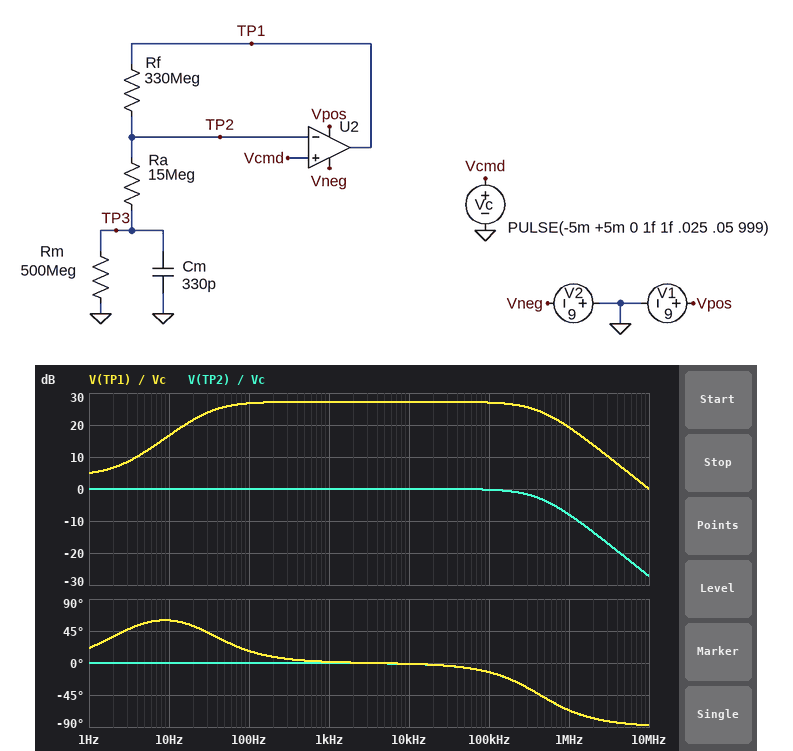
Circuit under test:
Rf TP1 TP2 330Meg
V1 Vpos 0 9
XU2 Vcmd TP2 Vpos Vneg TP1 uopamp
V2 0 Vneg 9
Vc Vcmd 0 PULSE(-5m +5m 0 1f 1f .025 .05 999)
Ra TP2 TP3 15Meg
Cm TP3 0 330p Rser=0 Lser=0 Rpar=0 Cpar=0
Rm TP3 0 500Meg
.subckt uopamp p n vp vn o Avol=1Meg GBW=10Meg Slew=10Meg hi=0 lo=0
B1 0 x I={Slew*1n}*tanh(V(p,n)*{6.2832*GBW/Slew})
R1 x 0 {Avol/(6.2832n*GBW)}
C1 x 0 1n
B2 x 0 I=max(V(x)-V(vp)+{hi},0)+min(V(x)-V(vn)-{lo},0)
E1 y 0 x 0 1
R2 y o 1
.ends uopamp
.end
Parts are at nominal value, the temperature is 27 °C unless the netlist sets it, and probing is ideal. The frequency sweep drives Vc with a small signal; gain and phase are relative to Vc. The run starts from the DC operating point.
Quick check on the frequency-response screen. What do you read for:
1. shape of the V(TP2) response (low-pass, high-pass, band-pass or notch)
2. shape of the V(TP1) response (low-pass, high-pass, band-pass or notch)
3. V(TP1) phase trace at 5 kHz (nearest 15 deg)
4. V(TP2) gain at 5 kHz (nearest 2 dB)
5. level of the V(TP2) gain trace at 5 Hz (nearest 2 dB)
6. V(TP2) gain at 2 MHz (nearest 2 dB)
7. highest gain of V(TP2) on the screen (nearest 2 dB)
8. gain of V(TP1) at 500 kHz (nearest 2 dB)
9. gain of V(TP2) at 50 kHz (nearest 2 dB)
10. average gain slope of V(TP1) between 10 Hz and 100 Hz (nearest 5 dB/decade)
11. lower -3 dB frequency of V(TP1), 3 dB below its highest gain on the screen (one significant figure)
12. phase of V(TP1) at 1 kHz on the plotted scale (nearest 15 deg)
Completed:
low-pass
band-pass
0 deg
0 dB
0 dB
-14 dB
0 dB
24 dB
0 dB
10 dB/decade
30 Hz
0 deg
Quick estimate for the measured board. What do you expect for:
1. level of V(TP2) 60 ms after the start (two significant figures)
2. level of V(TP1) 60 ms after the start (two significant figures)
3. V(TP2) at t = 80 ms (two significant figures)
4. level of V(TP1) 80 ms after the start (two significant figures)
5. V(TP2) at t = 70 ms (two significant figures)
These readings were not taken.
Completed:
5.0 mV
35 mV
-5.0 mV
-83 mV
5.0 mV
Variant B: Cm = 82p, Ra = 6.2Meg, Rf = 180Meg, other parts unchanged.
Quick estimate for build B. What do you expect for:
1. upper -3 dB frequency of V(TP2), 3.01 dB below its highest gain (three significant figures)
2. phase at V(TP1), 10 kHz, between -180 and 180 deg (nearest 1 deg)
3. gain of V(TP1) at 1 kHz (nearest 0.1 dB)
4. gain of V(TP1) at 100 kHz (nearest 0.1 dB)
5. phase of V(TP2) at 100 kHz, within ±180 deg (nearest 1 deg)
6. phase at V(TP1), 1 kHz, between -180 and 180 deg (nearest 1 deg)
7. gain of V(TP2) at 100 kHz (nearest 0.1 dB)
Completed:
333 kHz
0 deg
29.1 dB
29.2 dB
-17 deg
17 deg
-0.4 dB
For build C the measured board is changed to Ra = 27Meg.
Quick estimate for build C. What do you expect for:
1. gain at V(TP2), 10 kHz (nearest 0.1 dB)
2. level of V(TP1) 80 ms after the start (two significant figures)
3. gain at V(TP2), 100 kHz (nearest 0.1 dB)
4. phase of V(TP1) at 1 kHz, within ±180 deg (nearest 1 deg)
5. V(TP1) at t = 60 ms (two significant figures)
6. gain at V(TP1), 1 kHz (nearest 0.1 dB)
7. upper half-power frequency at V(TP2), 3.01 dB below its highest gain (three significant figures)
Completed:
0 dB
-69 mV
-0.1 dB
1 deg
42 mV
22.4 dB
756 kHz
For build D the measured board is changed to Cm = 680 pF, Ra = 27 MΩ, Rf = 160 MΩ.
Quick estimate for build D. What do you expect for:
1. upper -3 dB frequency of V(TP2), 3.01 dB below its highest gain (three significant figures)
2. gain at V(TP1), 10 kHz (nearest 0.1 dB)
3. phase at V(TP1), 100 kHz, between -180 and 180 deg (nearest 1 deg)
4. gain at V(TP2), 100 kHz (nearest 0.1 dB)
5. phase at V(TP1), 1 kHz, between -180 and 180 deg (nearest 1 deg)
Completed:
1.44 MHz
16.8 dB
-4 deg
0 dB
0 deg
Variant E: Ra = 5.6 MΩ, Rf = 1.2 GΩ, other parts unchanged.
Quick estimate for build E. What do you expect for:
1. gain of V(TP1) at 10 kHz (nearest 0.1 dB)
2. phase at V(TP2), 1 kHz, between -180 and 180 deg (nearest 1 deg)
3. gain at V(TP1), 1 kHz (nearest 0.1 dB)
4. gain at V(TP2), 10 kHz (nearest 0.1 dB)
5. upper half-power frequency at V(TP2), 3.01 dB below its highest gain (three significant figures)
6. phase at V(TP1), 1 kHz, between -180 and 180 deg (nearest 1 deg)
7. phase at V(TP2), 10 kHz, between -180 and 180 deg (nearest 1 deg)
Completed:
46.5 dB
-1 deg
46.6 dB
-0.2 dB
46.4 kHz
4 deg
-12 deg
